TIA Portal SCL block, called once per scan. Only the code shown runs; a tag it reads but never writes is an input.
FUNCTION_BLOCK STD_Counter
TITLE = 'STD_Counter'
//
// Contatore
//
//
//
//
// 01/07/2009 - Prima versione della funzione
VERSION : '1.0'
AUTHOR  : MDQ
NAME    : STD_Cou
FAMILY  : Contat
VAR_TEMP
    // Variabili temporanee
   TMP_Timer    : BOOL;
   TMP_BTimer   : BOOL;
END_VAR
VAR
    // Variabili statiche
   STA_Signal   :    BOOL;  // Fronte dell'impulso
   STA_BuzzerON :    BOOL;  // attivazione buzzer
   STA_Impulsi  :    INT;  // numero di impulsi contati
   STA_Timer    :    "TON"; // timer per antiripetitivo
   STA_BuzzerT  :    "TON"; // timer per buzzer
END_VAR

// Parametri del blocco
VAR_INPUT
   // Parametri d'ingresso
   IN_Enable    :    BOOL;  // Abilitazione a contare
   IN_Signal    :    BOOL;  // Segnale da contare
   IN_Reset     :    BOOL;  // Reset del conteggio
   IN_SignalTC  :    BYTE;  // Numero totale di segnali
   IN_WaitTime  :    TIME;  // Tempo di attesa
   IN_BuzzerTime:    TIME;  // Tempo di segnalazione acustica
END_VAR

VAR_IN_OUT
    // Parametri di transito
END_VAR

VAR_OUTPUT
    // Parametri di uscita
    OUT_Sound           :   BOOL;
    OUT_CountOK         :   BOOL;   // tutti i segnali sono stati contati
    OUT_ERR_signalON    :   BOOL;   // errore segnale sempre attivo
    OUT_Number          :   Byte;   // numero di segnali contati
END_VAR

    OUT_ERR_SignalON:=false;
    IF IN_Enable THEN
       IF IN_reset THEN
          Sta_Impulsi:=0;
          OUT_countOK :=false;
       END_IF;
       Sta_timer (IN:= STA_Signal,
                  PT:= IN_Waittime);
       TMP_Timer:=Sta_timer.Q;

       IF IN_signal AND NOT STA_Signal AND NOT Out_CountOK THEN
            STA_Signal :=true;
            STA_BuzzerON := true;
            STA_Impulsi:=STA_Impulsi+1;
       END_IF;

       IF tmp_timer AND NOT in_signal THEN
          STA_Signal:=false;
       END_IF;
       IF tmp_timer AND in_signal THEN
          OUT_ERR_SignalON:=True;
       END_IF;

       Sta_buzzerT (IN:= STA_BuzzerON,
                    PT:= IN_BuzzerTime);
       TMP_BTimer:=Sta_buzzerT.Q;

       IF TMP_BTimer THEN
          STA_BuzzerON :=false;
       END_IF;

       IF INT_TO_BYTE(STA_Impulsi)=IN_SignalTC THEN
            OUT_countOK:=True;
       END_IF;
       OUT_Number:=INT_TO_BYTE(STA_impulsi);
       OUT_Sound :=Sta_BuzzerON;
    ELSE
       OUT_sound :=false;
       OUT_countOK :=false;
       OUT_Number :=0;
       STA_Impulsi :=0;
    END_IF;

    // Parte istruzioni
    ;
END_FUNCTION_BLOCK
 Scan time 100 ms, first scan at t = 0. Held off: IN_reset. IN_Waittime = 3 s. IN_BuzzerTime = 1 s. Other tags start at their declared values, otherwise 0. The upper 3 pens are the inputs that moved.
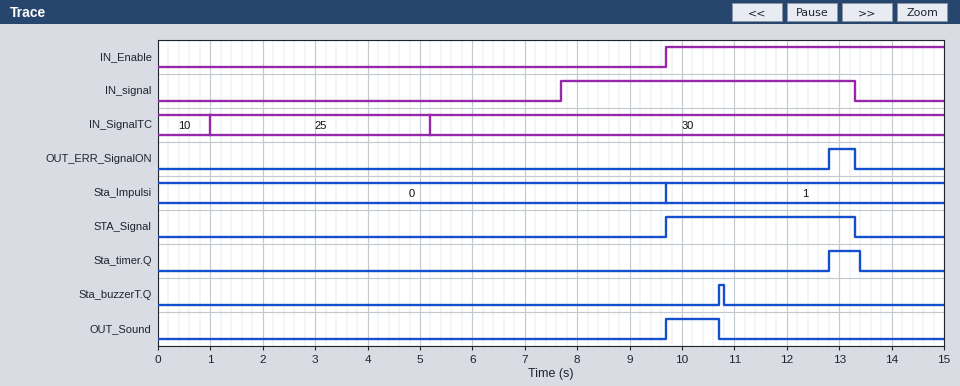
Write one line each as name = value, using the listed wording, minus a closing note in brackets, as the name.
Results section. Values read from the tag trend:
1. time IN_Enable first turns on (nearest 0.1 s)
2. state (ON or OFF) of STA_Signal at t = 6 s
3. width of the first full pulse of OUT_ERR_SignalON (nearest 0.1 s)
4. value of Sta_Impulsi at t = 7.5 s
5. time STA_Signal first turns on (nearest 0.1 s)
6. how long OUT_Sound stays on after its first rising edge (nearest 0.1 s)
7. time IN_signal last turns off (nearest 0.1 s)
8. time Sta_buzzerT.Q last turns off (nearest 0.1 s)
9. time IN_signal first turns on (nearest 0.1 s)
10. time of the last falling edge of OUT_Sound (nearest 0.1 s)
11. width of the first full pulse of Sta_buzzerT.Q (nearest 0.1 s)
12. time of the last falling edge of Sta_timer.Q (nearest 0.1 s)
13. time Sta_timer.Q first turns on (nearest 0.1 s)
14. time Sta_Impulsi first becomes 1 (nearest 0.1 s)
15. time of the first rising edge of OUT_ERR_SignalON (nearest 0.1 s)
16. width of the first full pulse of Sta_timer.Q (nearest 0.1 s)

time IN_Enable first turns on = 9.7 s
state (ON or OFF) of STA_Signal at t = 6 s = OFF
width of the first full pulse of OUT_ERR_SignalON = 0.5 s
value of Sta_Impulsi at t = 7.5 s = 0
time STA_Signal first turns on = 9.7 s
how long OUT_Sound stays on after its first rising edge = 1.0 s
time IN_signal last turns off = 13.3 s
time Sta_buzzerT.Q last turns off = 10.8 s
time IN_signal first turns on = 7.7 s
time of the last falling edge of OUT_Sound = 10.7 s
width of the first full pulse of Sta_buzzerT.Q = 0.1 s
time of the last falling edge of Sta_timer.Q = 13.4 s
time Sta_timer.Q first turns on = 12.8 s
time Sta_Impulsi first becomes 1 = 9.7 s
time of the first rising edge of OUT_ERR_SignalON = 12.8 s
width of the first full pulse of Sta_timer.Q = 0.6 s
